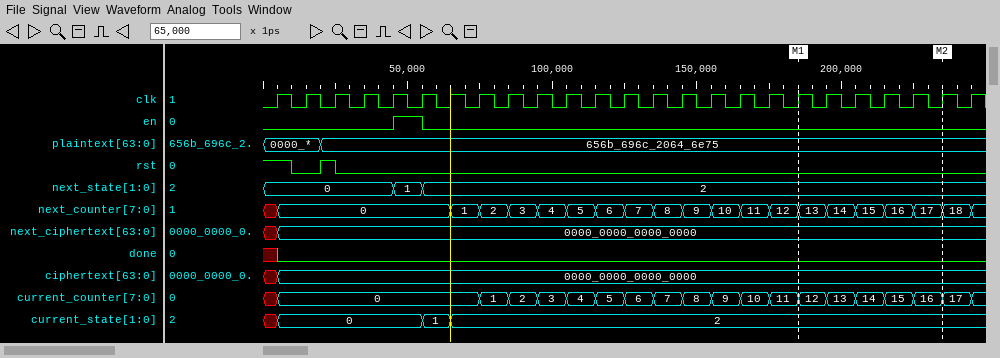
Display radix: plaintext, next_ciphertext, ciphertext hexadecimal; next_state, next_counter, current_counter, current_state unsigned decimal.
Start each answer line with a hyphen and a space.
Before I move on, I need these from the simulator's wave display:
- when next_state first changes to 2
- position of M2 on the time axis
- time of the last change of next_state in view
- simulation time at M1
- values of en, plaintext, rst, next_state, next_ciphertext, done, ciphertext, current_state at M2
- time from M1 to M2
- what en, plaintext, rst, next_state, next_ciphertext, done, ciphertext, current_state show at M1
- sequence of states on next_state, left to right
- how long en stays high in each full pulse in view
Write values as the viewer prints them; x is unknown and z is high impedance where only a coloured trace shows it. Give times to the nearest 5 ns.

- 55 ns
- 235 ns
- 55 ns
- 185 ns
- en=0, plaintext=656b_696c_2064_6e75, rst=0, next_state=2, next_ciphertext=0000_0000_0000_0000, done=0, ciphertext=0000_0000_0000_0000, current_state=2
- 50 ns
- en=0, plaintext=656b_696c_2064_6e75, rst=0, next_state=2, next_ciphertext=0000_0000_0000_0000, done=0, ciphertext=0000_0000_0000_0000, current_state=2
- 0, 1, 2
- 10 ns
